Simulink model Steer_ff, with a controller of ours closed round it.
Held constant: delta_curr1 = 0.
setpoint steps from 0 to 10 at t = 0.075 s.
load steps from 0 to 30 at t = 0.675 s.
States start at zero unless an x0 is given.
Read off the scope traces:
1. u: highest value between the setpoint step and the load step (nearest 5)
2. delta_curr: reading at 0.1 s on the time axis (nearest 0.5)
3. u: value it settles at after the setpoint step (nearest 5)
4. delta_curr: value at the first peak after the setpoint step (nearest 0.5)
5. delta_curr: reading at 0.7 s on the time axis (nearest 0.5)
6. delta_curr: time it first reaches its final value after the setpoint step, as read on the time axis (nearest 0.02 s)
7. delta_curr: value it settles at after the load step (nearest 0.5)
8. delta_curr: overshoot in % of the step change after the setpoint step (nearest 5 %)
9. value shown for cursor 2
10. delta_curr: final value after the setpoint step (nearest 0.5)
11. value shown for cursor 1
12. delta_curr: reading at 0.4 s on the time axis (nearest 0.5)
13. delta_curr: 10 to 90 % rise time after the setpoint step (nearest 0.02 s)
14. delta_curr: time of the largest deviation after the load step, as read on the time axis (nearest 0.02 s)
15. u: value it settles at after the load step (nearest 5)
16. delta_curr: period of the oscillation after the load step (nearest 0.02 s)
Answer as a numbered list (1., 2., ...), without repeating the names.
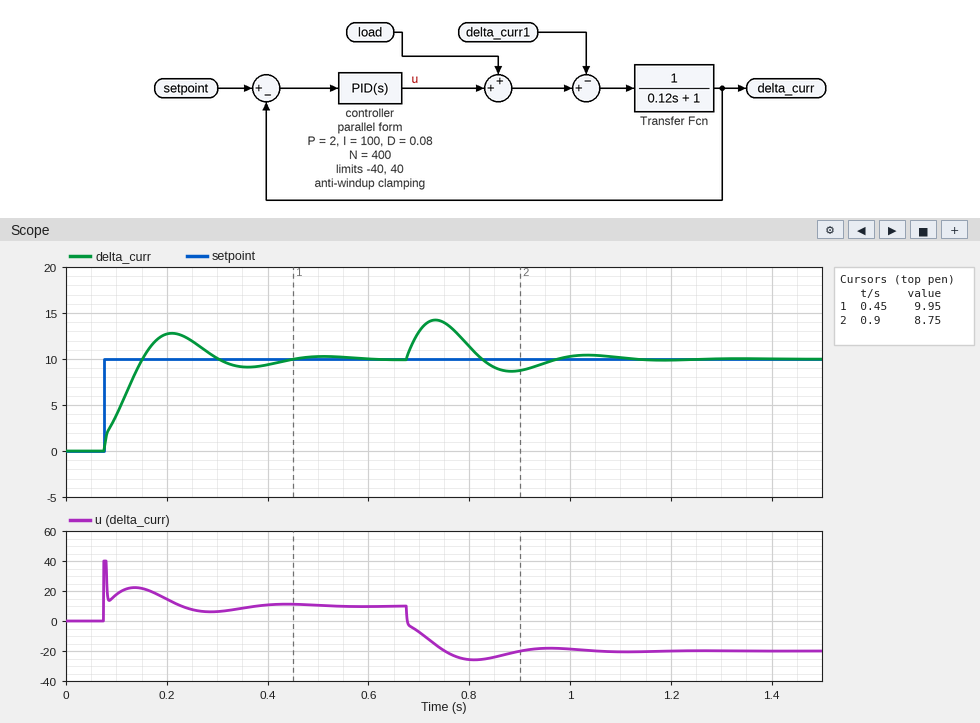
1. 40
2. 4.0
3. 10
4. 13.0
5. 13.0
6. 0.16 s
7. 10.0
8. 30 %
9. 8.75
10. 10.0
11. 9.95
12. 9.5
13. 0.06 s
14. 0.74 s
15. -20
16. 0.30 s
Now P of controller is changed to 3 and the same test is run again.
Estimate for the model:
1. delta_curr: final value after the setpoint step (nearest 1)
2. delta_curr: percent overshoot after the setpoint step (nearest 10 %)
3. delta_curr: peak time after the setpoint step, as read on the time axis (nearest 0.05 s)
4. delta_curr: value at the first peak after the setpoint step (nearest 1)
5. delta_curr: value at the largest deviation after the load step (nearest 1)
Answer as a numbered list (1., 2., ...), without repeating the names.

1. 10
2. 20 %
3. 0.20 s
4. 12
5. 14
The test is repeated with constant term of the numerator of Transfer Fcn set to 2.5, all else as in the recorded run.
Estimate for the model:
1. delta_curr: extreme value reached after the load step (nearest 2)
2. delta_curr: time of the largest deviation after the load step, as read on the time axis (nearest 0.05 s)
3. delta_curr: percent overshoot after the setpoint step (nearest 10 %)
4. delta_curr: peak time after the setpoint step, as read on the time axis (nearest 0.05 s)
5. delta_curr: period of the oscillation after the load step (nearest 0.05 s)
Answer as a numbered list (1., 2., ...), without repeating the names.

1. 16
2. 0.70 s
3. 20 %
4. 0.20 s
5. 0.25 s
